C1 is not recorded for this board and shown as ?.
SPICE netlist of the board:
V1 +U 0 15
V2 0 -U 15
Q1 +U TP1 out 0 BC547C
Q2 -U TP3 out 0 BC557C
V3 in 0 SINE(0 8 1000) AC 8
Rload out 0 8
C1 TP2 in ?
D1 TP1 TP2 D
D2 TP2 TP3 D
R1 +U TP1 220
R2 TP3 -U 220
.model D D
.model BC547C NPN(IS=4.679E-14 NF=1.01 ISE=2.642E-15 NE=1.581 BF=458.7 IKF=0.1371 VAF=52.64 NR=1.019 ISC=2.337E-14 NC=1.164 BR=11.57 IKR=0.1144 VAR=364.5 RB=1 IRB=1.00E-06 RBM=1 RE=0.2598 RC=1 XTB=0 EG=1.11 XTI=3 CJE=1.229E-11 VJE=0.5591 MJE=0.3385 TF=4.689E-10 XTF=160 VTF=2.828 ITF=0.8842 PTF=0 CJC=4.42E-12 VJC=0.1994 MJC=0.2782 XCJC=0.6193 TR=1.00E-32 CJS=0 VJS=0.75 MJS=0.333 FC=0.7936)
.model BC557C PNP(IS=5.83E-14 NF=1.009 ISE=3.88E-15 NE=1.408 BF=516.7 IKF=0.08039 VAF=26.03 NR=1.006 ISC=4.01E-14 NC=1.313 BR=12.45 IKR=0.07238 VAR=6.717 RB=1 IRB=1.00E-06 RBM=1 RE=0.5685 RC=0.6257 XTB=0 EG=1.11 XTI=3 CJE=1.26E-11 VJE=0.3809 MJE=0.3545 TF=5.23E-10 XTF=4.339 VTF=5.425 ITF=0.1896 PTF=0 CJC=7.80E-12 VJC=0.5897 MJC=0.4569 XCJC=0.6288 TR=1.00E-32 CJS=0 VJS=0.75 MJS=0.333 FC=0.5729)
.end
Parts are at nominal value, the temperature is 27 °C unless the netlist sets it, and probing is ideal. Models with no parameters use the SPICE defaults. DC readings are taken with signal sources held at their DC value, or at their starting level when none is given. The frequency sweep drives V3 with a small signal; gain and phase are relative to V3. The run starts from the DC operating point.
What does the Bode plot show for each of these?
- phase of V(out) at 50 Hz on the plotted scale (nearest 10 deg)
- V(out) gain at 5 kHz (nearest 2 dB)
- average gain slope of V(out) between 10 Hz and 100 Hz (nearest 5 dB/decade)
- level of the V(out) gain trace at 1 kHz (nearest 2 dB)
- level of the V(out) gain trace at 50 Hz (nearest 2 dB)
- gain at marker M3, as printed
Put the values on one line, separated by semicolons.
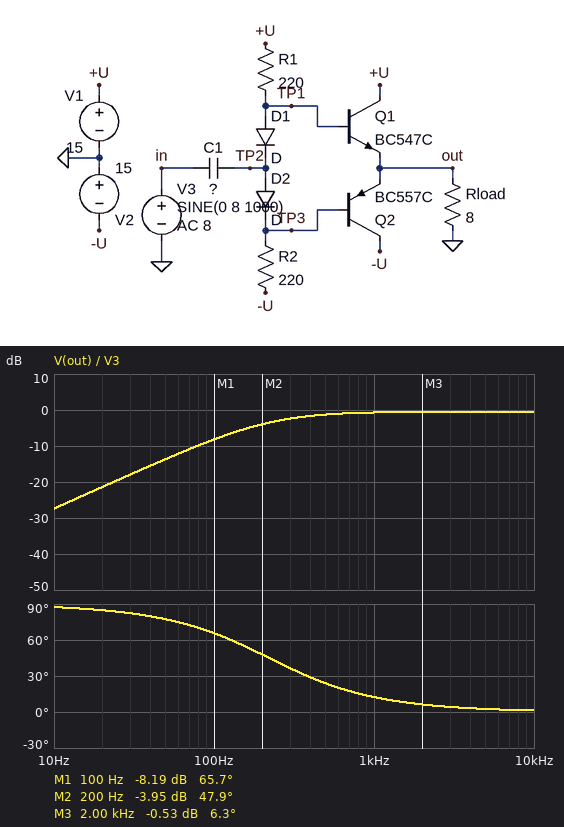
80 deg; 0 dB; 20 dB/decade; 0 dB; -14 dB; -0.53 dB
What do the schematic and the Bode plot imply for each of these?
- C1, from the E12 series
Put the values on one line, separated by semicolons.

6.8 µF
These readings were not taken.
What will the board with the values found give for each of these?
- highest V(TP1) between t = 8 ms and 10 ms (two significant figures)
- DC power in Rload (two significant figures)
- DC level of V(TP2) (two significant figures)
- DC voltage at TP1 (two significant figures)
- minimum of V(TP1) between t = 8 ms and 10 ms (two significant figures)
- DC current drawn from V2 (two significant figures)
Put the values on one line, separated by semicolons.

8.6 V; 4.1 µW; -2.0 mV; 760 mV; -6.9 V; 140 mA
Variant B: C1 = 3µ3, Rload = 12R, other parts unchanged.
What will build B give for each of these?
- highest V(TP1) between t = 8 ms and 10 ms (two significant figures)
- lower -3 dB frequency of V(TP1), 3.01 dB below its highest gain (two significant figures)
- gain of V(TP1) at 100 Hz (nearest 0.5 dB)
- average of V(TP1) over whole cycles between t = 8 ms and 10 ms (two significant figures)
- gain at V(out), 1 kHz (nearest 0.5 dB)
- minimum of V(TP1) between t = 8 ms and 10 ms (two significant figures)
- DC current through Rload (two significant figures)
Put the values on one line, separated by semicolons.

8.0 V; 450 Hz; -13.5 dB; 790 mV; -1.0 dB; -6.4 V; 490 µA
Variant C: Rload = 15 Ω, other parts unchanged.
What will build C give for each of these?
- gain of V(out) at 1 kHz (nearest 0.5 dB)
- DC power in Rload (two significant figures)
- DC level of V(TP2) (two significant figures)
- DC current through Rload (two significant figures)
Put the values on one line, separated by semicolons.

-0.5 dB; 2.4 µW; -1.9 mV; 400 µA
